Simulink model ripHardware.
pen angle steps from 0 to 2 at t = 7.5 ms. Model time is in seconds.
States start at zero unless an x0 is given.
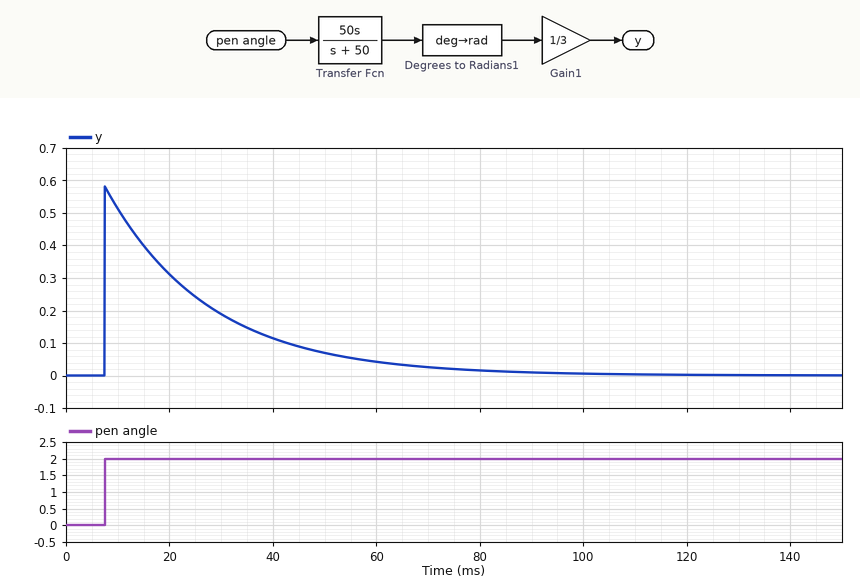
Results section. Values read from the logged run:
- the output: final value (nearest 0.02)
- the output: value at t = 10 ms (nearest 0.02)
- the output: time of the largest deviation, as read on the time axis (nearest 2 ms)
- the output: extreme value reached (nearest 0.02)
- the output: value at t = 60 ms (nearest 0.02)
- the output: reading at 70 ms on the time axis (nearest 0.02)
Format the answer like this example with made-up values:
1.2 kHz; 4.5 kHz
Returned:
0.00; 0.52; 8 ms; 0.58; 0.04; 0.02
